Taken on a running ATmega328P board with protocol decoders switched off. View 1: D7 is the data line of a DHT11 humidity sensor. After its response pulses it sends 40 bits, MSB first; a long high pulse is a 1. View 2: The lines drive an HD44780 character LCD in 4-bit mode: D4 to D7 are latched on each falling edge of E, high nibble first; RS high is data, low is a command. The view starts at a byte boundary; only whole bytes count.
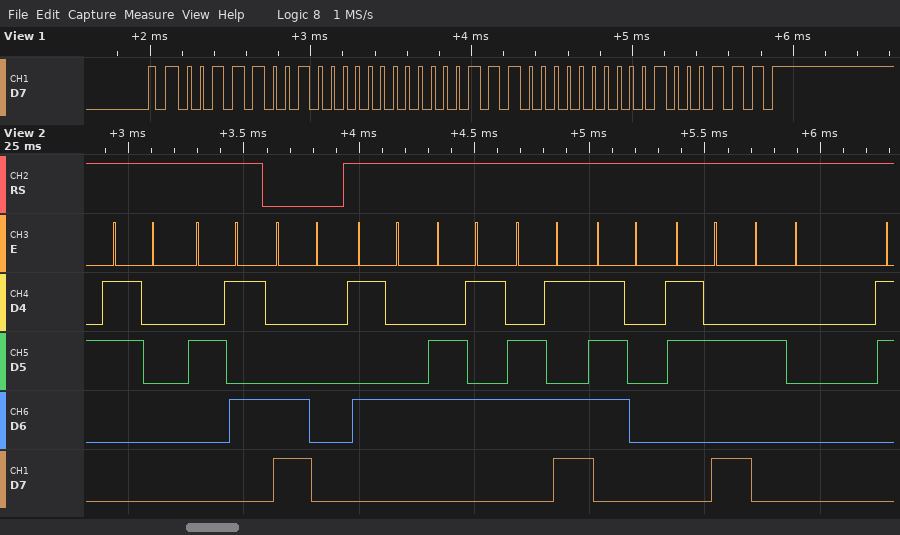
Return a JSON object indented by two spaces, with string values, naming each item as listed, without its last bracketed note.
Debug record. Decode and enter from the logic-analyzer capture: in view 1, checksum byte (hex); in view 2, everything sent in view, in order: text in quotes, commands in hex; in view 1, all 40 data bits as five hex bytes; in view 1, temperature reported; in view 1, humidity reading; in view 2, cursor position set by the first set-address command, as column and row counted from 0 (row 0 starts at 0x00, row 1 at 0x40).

{
  "in view 1, checksum byte": "0x47",
  "in view 2, everything sent in view, in order: text in quotes, commands in hex": "\"0%\" 0xC0 \"Temp: \"",
  "in view 1, all 40 data bits as five hex bytes": "39 00 0E 00 47",
  "in view 1, temperature reported": "14.0 °C",
  "in view 1, humidity reading": "57 %",
  "in view 2, cursor position set by the first set-address command, as column and row counted from 0": "column 0, row 1"
}
